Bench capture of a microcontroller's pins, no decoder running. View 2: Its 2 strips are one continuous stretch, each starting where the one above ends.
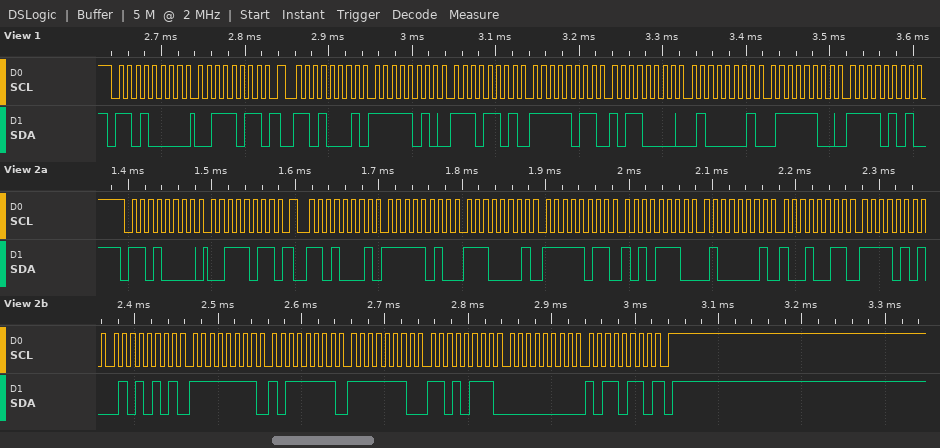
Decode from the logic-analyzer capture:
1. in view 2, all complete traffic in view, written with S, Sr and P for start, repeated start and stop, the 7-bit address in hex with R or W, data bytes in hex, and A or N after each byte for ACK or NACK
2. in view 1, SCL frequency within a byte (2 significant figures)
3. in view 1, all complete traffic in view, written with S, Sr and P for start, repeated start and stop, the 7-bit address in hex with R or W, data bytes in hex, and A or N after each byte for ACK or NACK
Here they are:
S 68W A 3B A Sr 68R A FA A E1 A FB A AE A 41 A 93 A F5 A 55 A FF A BF A FE A D7 A 00 A B6 N P
100 kHz
S 68W A 3B A Sr 68R A FA A ED A FB A B0 A 41 A 7C A F5 A
